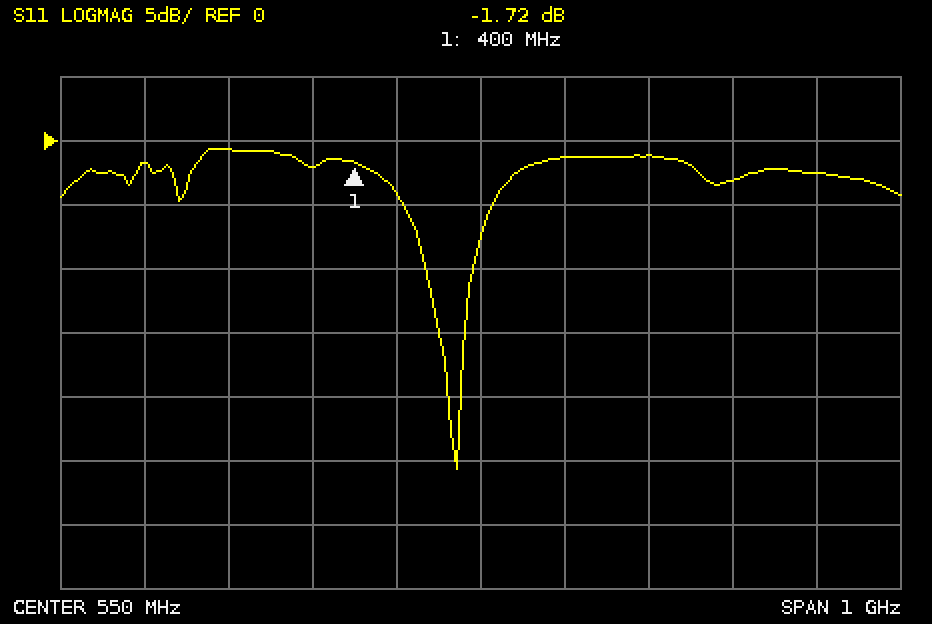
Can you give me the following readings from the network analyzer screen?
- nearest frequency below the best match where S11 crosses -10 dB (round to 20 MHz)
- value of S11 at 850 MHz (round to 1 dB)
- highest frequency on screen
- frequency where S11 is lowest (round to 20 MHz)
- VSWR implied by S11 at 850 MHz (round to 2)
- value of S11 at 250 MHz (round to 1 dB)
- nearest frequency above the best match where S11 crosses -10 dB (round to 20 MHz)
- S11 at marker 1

480 MHz
-3 dB
1.05 GHz
520 MHz
6
-1 dB
540 MHz
-1.72 dB
